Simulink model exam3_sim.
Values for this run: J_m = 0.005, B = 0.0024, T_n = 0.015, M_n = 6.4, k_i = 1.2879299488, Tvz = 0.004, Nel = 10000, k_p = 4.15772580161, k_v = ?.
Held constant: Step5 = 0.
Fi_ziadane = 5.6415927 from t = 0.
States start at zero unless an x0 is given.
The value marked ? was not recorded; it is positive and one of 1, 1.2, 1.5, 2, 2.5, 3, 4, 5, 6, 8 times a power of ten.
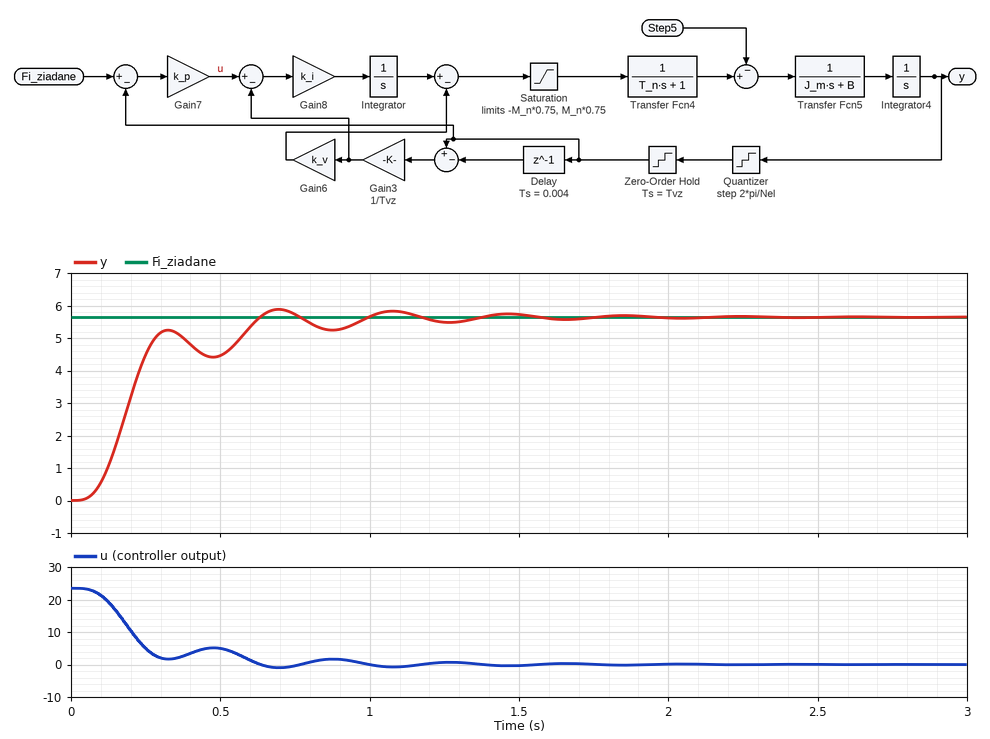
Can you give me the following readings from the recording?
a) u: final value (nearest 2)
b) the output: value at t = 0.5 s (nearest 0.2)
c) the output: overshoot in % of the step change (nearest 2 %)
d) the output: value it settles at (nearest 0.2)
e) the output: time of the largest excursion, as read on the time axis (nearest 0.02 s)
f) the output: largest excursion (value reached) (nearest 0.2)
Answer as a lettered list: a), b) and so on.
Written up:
a) 0
b) 4.4
c) 4 %
d) 5.6
e) 0.70 s
f) 5.8
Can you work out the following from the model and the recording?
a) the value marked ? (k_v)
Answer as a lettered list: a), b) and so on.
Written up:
a) 0.06
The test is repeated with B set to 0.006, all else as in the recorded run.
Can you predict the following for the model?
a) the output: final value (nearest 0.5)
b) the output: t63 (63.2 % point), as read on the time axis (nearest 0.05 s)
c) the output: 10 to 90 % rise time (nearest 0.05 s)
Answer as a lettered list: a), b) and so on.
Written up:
a) 5.5
b) 0.20 s
c) 0.20 s
